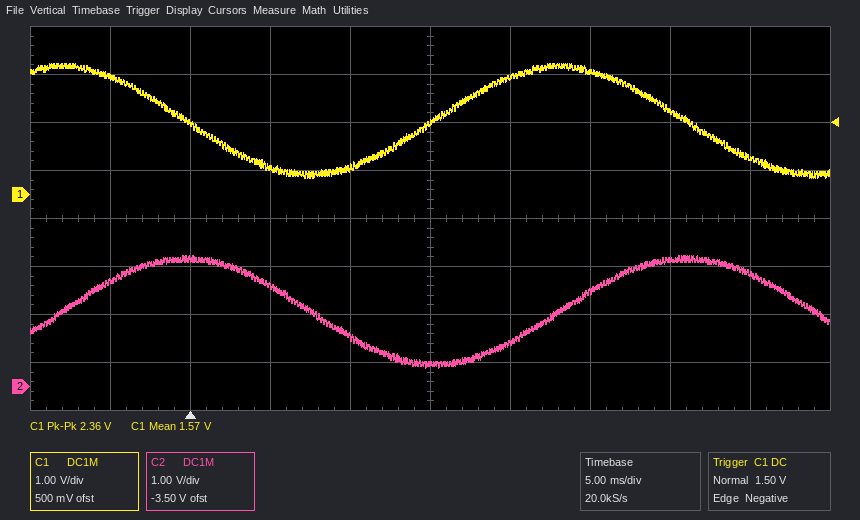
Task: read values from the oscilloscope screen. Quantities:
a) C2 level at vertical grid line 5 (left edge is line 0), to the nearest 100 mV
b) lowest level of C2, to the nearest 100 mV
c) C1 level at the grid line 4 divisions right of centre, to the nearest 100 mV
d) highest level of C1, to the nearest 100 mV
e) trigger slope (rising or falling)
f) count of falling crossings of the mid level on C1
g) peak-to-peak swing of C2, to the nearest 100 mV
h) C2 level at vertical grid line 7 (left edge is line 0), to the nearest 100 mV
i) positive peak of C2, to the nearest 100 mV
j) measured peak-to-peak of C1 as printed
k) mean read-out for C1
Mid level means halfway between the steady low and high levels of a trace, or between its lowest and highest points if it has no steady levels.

500 mV
400 mV
800 mV
2.7 V
falling
2
2.3 V
2.0 V
2.7 V
2.36 V
1.57 V
